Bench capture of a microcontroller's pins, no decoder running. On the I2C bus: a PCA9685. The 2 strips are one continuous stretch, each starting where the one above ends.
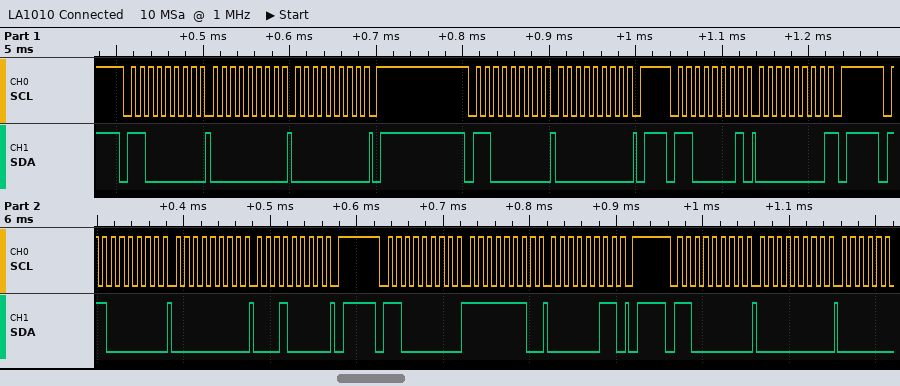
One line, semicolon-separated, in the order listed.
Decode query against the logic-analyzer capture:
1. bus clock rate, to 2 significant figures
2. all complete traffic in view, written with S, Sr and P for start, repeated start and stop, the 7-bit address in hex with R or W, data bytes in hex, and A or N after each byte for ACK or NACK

100 kHz; S 60W A 00 A 00 A P S 60W A 00 A P S 60R A 00 N P S 60W A 00 A 10 A P S 60W A FE A 03 A P S 60W A 00 A
